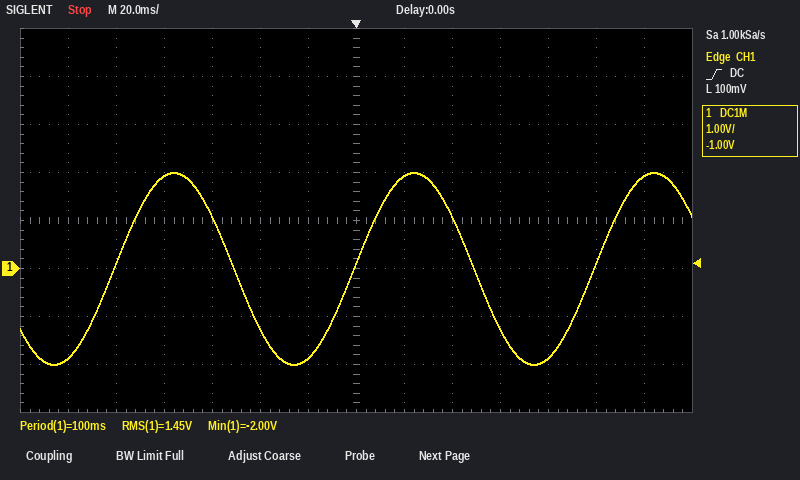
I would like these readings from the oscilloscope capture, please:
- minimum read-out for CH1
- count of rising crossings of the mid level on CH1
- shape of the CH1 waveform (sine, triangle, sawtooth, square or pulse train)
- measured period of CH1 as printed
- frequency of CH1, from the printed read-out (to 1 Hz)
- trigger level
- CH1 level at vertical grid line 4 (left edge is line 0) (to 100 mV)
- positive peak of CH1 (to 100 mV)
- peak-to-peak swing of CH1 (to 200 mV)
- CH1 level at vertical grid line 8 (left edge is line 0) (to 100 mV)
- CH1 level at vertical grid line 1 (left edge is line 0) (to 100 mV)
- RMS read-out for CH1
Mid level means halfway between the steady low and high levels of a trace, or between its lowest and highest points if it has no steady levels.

-2.00 V
3
sine
100 ms
10 Hz
100 mV
1.1 V
2.0 V
4.0 V
1.9 V
-1.9 V
1.45 V
